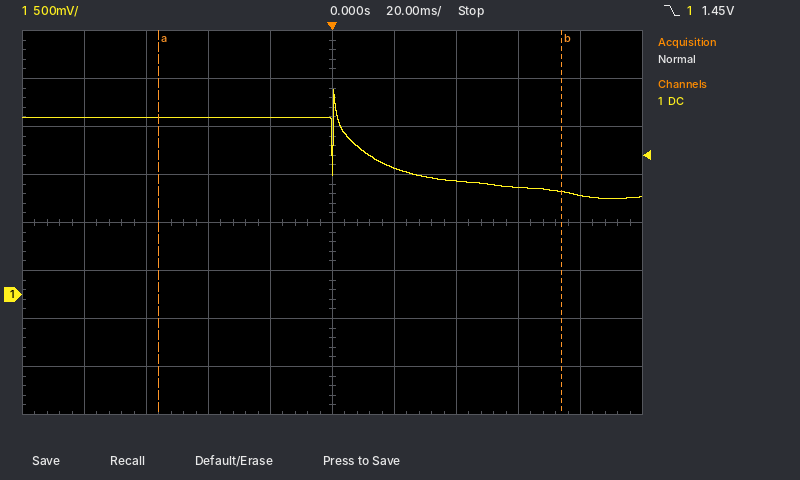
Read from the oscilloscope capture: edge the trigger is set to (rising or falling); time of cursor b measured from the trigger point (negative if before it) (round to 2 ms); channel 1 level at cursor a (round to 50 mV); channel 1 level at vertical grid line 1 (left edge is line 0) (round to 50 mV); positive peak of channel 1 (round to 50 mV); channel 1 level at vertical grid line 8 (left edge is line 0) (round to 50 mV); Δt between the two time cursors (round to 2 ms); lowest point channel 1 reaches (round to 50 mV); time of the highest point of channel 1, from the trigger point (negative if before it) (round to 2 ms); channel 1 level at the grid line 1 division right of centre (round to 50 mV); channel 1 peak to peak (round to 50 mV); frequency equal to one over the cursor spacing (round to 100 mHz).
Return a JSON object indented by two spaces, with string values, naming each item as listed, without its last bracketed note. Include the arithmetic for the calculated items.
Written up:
{
  "edge the trigger is set to": "falling",
  "time of cursor b measured from the trigger point (negative if before it)": "+74 ms",
  "channel 1 level at cursor a": "1.85 V",
  "channel 1 level at vertical grid line 1 (left edge is line 0)": "1.85 V",
  "positive peak of channel 1": "2.15 V",
  "channel 1 level at vertical grid line 8 (left edge is line 0)": "1.10 V",
  "Δt between the two time cursors": "130 ms",
  "lowest point channel 1 reaches": "1.00 V",
  "time of the highest point of channel 1, from the trigger point (negative if before it)": "0 ms",
  "channel 1 level at the grid line 1 division right of centre": "1.30 V",
  "channel 1 peak to peak": "2.15 V − (1.00 V) = 1.15 V",
  "frequency equal to one over the cursor spacing": "1 / 130 ms ≈ 7.7 Hz"
}
